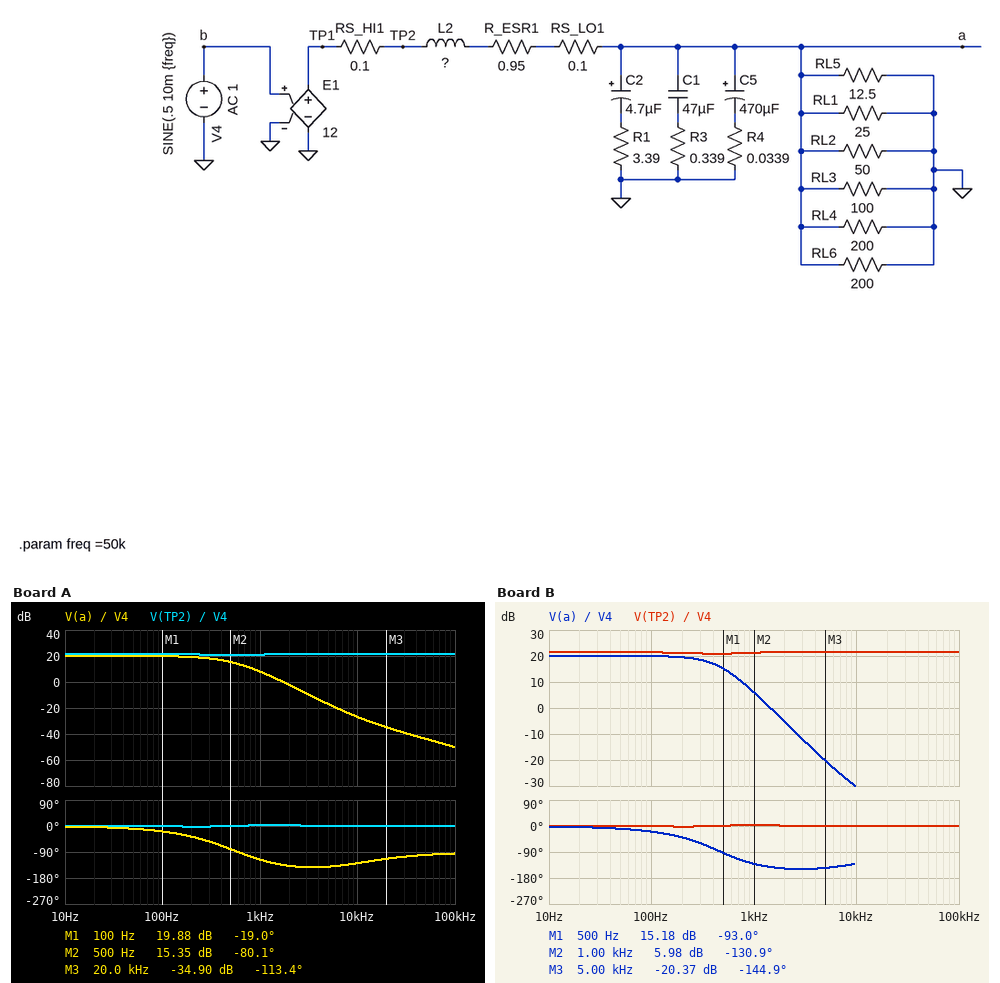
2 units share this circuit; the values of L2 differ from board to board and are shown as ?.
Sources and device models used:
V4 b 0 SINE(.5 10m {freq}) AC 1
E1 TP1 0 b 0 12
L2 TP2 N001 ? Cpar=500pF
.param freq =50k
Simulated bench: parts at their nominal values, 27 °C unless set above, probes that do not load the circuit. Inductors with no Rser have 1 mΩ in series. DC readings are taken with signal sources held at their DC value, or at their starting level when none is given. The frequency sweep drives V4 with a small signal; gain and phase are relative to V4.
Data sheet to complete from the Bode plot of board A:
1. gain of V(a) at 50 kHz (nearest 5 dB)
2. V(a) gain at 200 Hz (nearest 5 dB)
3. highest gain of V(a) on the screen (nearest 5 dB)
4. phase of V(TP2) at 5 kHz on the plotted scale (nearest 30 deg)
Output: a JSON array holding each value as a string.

["-45 dB", "20 dB", "20 dB", "0 deg"]
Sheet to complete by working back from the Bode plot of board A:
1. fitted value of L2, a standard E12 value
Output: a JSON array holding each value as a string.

["180 µH"]
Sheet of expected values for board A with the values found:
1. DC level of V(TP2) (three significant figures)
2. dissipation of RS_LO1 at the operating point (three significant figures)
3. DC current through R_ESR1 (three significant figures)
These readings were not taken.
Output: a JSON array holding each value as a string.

["5.92 V", "65.7 mW", "811 mA"]
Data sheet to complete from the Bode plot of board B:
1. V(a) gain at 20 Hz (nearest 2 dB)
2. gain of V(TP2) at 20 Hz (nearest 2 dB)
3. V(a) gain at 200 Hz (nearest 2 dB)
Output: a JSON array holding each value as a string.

["20 dB", "22 dB", "20 dB"]
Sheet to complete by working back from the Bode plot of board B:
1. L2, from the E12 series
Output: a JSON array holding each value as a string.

["270 µH"]
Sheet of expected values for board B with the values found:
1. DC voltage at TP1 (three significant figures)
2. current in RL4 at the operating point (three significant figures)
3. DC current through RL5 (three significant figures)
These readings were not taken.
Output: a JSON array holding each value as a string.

["6.00 V", "25.3 mA", "405 mA"]
